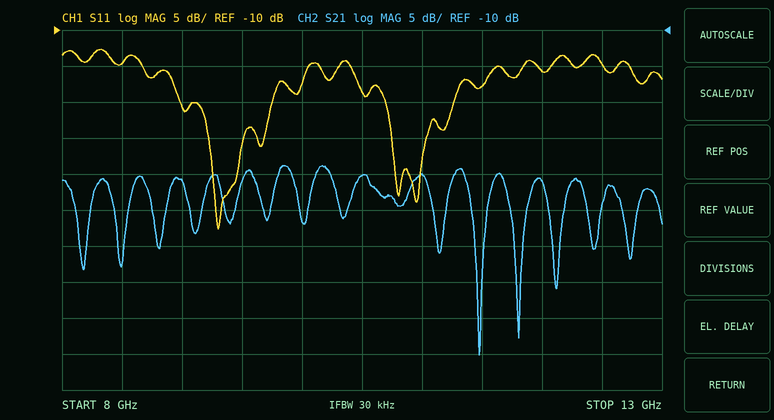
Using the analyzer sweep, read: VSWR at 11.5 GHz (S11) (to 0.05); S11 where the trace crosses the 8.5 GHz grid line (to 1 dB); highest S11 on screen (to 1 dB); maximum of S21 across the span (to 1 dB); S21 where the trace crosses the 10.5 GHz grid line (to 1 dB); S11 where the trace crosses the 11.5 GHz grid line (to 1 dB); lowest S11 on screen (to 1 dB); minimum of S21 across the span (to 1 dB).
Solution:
1.30
-15 dB
-13 dB
-29 dB
-30 dB
-18 dB
-38 dB
-55 dB
